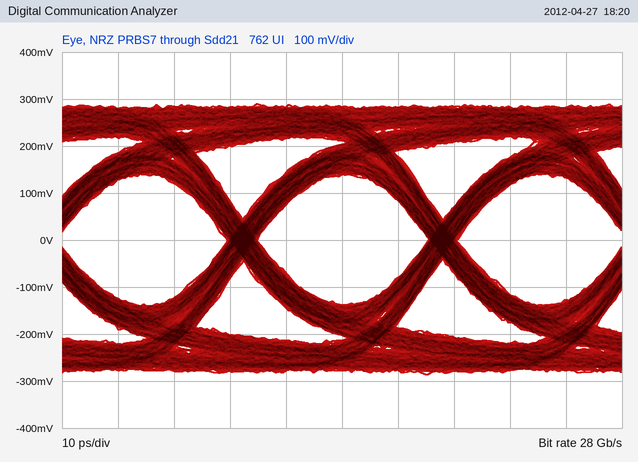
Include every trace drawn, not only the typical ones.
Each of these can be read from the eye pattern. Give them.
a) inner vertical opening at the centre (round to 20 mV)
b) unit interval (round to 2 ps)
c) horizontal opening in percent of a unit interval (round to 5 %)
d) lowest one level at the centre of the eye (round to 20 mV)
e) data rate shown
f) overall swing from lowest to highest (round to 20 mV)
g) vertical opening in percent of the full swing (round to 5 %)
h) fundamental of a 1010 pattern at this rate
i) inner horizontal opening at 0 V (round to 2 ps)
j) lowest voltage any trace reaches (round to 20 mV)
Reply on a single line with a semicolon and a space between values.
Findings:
280 mV; 36 ps; 85 %; 140 mV; 28 Gb/s; 580 mV; 50 %; 14 GHz; 30 ps; -280 mV
